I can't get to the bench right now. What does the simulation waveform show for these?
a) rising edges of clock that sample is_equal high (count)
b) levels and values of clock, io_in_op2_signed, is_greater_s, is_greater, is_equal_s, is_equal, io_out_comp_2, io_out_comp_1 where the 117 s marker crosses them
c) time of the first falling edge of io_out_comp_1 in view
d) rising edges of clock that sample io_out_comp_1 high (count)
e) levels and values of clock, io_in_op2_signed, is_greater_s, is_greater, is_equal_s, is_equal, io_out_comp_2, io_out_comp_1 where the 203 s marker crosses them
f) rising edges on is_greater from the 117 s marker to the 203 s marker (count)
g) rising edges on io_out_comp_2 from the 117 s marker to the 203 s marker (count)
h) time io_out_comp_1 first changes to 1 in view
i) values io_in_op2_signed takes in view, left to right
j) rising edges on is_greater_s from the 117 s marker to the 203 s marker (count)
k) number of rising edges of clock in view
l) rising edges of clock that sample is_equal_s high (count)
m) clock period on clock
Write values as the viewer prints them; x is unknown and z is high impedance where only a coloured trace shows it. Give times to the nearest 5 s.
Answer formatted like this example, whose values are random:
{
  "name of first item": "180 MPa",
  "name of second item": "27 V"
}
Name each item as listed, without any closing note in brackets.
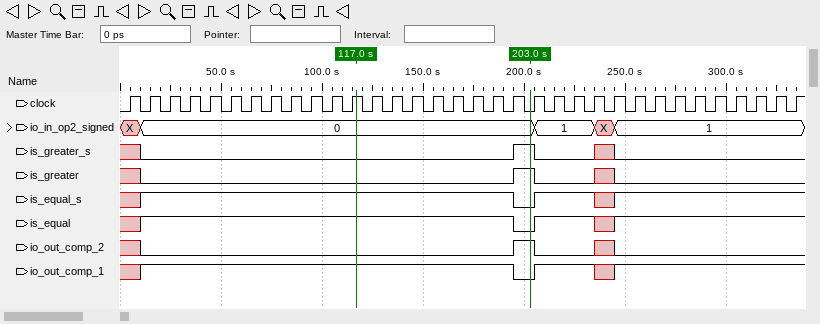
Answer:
{
  "rising edges of clock that sample is_equal high": "31",
  "levels and values of clock, io_in_op2_signed, is_greater_s, is_greater, is_equal_s, is_equal, io_out_comp_2, io_out_comp_1 where the 117 s marker crosses them": "clock=1, io_in_op2_signed=0, is_greater_s=0, is_greater=0, is_equal_s=1, is_equal=1, io_out_comp_2=0, io_out_comp_1=1",
  "time of the first falling edge of io_out_comp_1 in view": "195 s",
  "rising edges of clock that sample io_out_comp_1 high": "31",
  "levels and values of clock, io_in_op2_signed, is_greater_s, is_greater, is_equal_s, is_equal, io_out_comp_2, io_out_comp_1 where the 203 s marker crosses them": "clock=0, io_in_op2_signed=0, is_greater_s=1, is_greater=1, is_equal_s=0, is_equal=0, io_out_comp_2=1, io_out_comp_1=0",
  "rising edges on is_greater from the 117 s marker to the 203 s marker": "1",
  "rising edges on io_out_comp_2 from the 117 s marker to the 203 s marker": "1",
  "time io_out_comp_1 first changes to 1 in view": "10 s",
  "values io_in_op2_signed takes in view, left to right": "X, 0, 1, X, 1",
  "rising edges on is_greater_s from the 117 s marker to the 203 s marker": "1",
  "number of rising edges of clock in view": "34",
  "rising edges of clock that sample is_equal_s high": "31",
  "clock period on clock": "10 s"
}
